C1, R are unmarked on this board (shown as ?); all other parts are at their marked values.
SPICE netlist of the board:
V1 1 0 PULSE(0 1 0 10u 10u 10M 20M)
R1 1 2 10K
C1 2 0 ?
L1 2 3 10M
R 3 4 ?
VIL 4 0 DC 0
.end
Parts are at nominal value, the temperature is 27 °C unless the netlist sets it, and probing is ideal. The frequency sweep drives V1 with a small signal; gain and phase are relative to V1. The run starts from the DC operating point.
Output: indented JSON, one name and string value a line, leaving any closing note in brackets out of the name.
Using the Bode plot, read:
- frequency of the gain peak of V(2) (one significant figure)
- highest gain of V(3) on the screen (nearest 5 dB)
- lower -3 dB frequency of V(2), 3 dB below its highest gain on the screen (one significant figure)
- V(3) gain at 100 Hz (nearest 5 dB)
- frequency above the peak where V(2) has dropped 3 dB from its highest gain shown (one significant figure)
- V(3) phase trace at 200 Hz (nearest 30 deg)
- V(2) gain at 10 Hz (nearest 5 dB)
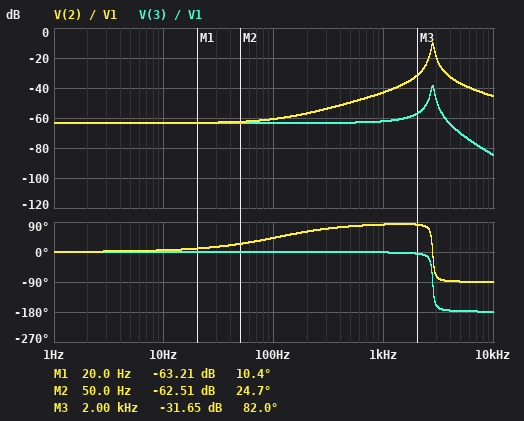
{
  "frequency of the gain peak of V(2)": "3 kHz",
  "highest gain of V(3) on the screen": "-40 dB",
  "lower -3 dB frequency of V(2), 3 dB below its highest gain on the screen": "3 kHz",
  "V(3) gain at 100 Hz": "-65 dB",
  "frequency above the peak where V(2) has dropped 3 dB from its highest gain shown": "3 kHz",
  "V(3) phase trace at 200 Hz": "0 deg",
  "V(2) gain at 10 Hz": "-65 dB"
}
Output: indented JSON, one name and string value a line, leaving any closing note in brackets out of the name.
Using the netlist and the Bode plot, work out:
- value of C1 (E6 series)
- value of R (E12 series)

{
  "value of C1": "330 nF",
  "value of R": "6.8 Ω"
}
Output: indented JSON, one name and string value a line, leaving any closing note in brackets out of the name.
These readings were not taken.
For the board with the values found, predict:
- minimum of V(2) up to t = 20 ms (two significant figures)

{
  "minimum of V(2) up to t = 20 ms": "-17 mV"
}
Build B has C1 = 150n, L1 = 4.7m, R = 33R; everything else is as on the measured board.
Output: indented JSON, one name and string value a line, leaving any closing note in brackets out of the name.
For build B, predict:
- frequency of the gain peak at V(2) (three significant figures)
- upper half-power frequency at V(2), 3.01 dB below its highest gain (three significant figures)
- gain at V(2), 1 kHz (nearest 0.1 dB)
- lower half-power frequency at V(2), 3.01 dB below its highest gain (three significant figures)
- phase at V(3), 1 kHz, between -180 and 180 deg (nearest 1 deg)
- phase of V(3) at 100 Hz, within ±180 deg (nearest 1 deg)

{
  "frequency of the gain peak at V(2)": "6.00 kHz",
  "upper half-power frequency at V(2), 3.01 dB below its highest gain": "6.64 kHz",
  "gain at V(2), 1 kHz": "-46.9 dB",
  "lower half-power frequency at V(2), 3.01 dB below its highest gain": "5.42 kHz",
  "phase at V(3), 1 kHz, between -180 and 180 deg": "-2 deg",
  "phase of V(3) at 100 Hz, within ±180 deg": "0 deg"
}
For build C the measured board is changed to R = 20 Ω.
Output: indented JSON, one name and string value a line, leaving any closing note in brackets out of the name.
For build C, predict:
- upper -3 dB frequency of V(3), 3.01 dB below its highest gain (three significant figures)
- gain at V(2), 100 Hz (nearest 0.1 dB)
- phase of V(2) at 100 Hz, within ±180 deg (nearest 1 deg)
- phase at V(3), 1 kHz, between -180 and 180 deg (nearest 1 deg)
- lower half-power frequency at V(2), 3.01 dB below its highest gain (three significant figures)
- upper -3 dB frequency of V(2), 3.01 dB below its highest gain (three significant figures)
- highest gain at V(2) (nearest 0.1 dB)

{
  "upper -3 dB frequency of V(3), 3.01 dB below its highest gain": "2.94 kHz",
  "gain at V(2), 100 Hz": "-53.6 dB",
  "phase of V(2) at 100 Hz, within ±180 deg": "17 deg",
  "phase at V(3), 1 kHz, between -180 and 180 deg": "-3 deg",
  "lower half-power frequency at V(2), 3.01 dB below its highest gain": "2.60 kHz",
  "upper -3 dB frequency of V(2), 3.01 dB below its highest gain": "2.96 kHz",
  "highest gain at V(2)": "-17.6 dB"
}
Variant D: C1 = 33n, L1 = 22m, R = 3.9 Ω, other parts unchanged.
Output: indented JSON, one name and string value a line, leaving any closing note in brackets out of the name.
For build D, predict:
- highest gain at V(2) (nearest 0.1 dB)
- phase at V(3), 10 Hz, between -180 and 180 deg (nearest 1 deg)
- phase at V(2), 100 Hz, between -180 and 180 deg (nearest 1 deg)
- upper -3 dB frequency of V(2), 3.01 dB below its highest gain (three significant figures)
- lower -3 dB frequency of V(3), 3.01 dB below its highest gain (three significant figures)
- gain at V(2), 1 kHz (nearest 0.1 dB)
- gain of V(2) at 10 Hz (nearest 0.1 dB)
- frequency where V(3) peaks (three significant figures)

{
  "highest gain at V(2)": "-0.5 dB",
  "phase at V(3), 10 Hz, between -180 and 180 deg": "0 deg",
  "phase at V(2), 100 Hz, between -180 and 180 deg": "74 deg",
  "upper -3 dB frequency of V(2), 3.01 dB below its highest gain": "6.17 kHz",
  "lower -3 dB frequency of V(3), 3.01 dB below its highest gain": "5.64 kHz",
  "gain at V(2), 1 kHz": "-36.9 dB",
  "gain of V(2) at 10 Hz": "-67.7 dB",
  "frequency where V(3) peaks": "5.90 kHz"
}
